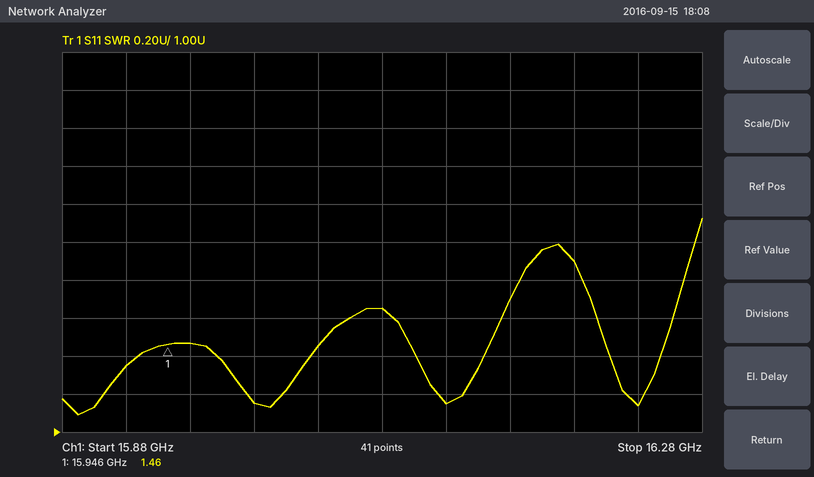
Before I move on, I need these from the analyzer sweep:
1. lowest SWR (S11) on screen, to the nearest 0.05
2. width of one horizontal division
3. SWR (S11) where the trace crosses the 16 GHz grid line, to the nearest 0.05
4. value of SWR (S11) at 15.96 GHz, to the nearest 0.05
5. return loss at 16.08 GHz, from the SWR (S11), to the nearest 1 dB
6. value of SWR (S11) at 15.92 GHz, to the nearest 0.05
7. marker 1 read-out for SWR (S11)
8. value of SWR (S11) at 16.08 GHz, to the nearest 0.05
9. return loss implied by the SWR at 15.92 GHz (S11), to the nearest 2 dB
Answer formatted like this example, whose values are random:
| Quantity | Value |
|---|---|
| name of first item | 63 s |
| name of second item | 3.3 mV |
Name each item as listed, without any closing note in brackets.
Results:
| Quantity | Value |
|---|---|
| lowest SWR (S11) on screen, to the nearest 0.05 | 1.10 |
| width of one horizontal division | 40 MHz |
| SWR (S11) where the trace crosses the 16 GHz grid line, to the nearest 0.05 | 1.15 |
| value of SWR (S11) at 15.96 GHz, to the nearest 0.05 | 1.45 |
| return loss at 16.08 GHz, from the SWR (S11), to the nearest 1 dB | 12 dB |
| value of SWR (S11) at 15.92 GHz, to the nearest 0.05 | 1.35 |
| marker 1 read-out for SWR | 1.46 |
| value of SWR (S11) at 16.08 GHz, to the nearest 0.05 | 1.65 |
| return loss implied by the SWR at 15.92 GHz (S11), to the nearest 2 dB | 16 dB |
